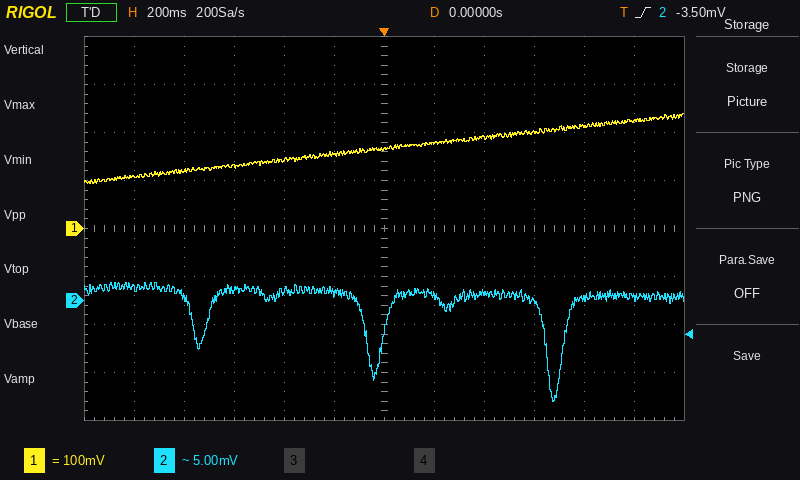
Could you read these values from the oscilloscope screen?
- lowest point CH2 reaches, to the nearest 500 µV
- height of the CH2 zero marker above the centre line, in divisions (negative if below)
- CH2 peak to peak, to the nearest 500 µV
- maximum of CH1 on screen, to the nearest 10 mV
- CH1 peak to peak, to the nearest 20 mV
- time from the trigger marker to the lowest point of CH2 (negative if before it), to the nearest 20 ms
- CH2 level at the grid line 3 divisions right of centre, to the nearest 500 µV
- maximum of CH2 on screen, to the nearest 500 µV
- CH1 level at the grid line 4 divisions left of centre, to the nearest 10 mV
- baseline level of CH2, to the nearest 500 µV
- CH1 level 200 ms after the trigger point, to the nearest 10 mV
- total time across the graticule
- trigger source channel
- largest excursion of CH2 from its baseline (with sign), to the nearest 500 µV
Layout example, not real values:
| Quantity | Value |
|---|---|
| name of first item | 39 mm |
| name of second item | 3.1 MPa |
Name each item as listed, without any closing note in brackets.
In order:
| Quantity | Value |
|---|---|
| lowest point CH2 reaches, to the nearest 500 µV | -10.5 mV |
| height of the CH2 zero marker above the centre line, in divisions | -1.5 div |
| CH2 peak to peak, to the nearest 500 µV | 12.5 mV |
| maximum of CH1 on screen, to the nearest 10 mV | 240 mV |
| CH1 peak to peak, to the nearest 20 mV | 140 mV |
| time from the trigger marker to the lowest point of CH2 (negative if before it), to the nearest 20 ms | +680 ms |
| CH2 level at the grid line 3 divisions right of centre, to the nearest 500 µV | 0.0 mV |
| maximum of CH2 on screen, to the nearest 500 µV | 2.0 mV |
| CH1 level at the grid line 4 divisions left of centre, to the nearest 10 mV | 120 mV |
| baseline level of CH2, to the nearest 500 µV | 500 µV |
| CH1 level 200 ms after the trigger point, to the nearest 10 mV | 180 mV |
| total time across the graticule | 2.4 s |
| trigger source channel | CH2 |
| largest excursion of CH2 from its baseline (with sign), to the nearest 500 µV | -11.0 mV |
